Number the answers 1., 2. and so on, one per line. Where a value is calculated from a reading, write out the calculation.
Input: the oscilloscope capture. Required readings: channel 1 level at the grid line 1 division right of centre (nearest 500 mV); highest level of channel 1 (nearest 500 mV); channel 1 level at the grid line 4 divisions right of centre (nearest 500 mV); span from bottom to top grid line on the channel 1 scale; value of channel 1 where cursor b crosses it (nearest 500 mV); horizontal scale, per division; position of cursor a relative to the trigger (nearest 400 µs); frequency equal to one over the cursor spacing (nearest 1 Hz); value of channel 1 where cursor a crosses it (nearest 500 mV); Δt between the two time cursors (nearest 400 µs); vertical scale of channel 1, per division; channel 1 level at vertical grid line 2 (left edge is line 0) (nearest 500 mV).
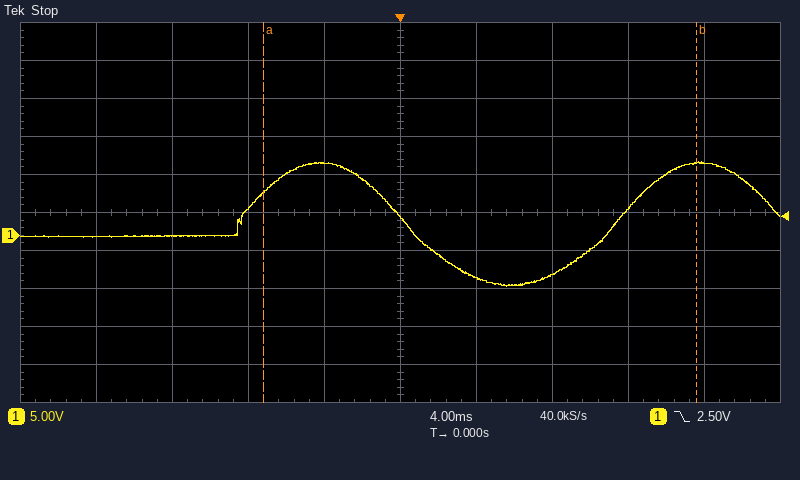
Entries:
1. -5.5 V
2. 9.5 V
3. 9.5 V
4. 50 V
5. 9.5 V
6. 4 ms
7. -7.2 ms
8. 1 / 22.8 ms ≈ 44 Hz
9. 5.5 V
10. 22.8 ms
11. 5 V
12. 0.0 V
